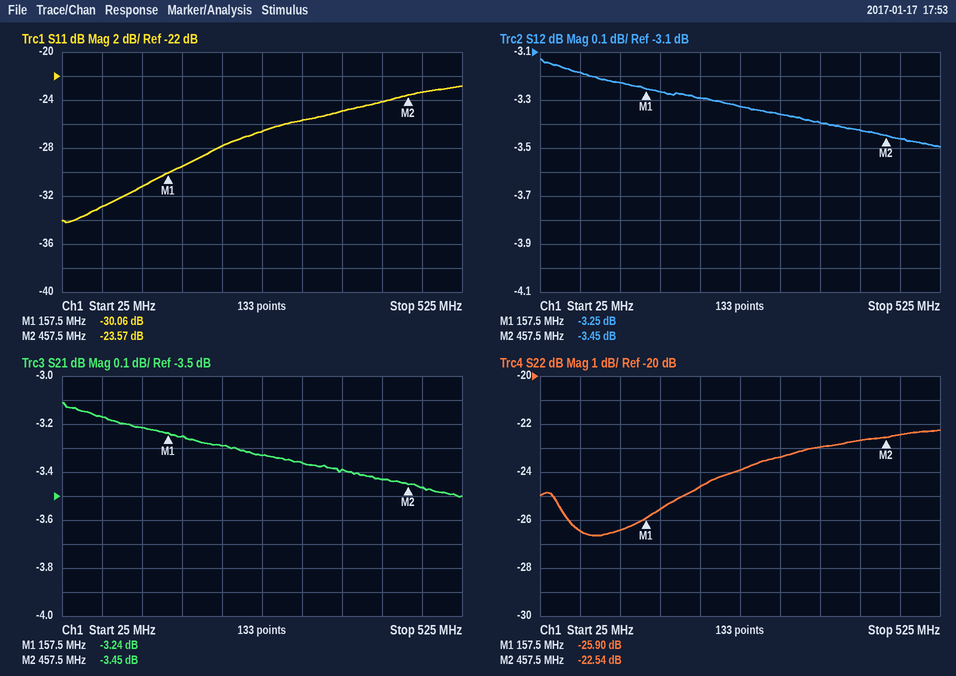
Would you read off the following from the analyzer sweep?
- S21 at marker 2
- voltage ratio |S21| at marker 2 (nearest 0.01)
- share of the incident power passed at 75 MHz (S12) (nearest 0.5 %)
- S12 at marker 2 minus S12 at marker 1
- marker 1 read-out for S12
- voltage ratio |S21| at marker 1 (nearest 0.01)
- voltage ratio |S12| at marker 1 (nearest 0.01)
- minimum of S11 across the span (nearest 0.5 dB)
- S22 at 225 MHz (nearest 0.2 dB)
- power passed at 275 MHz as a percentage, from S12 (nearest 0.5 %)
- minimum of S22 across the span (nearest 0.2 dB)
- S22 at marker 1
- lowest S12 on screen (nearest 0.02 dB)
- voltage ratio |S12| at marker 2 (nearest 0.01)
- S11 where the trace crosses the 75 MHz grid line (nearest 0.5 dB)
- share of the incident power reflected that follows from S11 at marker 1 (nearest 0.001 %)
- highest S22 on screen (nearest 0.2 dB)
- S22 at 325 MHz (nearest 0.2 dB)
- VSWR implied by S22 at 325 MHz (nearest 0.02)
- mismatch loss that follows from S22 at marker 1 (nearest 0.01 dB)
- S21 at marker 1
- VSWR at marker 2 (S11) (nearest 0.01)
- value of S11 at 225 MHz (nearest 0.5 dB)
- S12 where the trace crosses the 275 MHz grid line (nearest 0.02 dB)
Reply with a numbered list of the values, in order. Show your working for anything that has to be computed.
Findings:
1. -3.45 dB
2. 10^(-3.45/20) ≈ 0.67
3. 10^(-3.18/10) ≈ 48.1 %, so 48.0 % to the nearest 0.5 %
4. -3.45 − (-3.25) = -0.20 dB
5. -3.25 dB
6. 10^(-3.24/20) ≈ 0.69
7. 10^(-3.25/20) ≈ 0.69
8. -34.0 dB
9. -24.6 dB
10. 10^(-3.32/10) ≈ 46.6 %, so 46.5 % to the nearest 0.5 %
11. -26.6 dB
12. -25.90 dB
13. -3.50 dB
14. 10^(-3.45/20) ≈ 0.67
15. -33.0 dB
16. 10^(-30.06/10) ≈ 0.099 %
17. -22.2 dB
18. -23.4 dB
19. |Γ| = 10^(-23.4/20) = 0.0676; VSWR = (1 + 0.0676)/(1 − 0.0676) ≈ 1.15, so 1.14 to the nearest 0.02
20. −10 log10(1 − 10^(-25.9/10)) ≈ 0.01 dB
21. -3.24 dB
22. (1 + 0.0663)/(1 − 0.0663) ≈ 1.14
23. -28.0 dB
24. -3.32 dB
